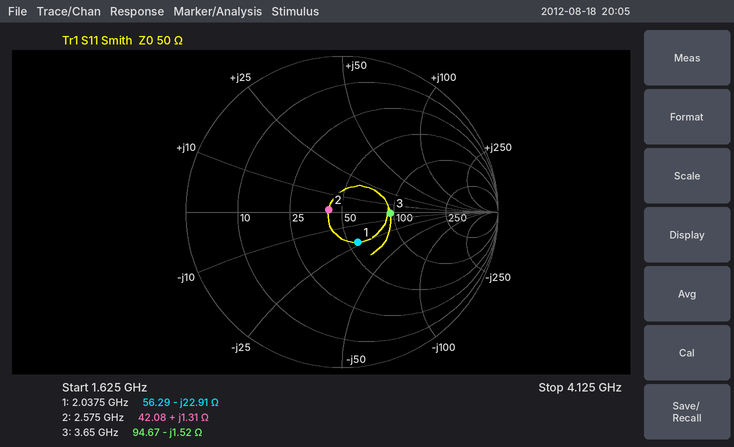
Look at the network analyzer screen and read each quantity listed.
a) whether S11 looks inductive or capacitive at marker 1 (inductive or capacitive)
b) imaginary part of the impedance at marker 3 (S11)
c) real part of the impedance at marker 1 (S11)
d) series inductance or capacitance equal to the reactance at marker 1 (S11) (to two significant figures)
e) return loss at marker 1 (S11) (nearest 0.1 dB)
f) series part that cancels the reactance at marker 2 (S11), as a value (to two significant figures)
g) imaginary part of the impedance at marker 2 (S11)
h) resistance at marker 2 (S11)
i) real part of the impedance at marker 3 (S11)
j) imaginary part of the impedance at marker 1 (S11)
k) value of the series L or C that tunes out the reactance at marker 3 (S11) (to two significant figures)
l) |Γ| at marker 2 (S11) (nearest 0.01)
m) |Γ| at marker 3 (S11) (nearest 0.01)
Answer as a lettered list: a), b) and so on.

a) capacitive
b) -1.52 Ω
c) 56.29 Ω
d) 3.4 pF
e) 13.2 dB
f) 47 pF
g) +1.31 Ω
h) 42.08 Ω
i) 94.67 Ω
j) -22.91 Ω
k) 66 pH
l) 0.09
m) 0.31
